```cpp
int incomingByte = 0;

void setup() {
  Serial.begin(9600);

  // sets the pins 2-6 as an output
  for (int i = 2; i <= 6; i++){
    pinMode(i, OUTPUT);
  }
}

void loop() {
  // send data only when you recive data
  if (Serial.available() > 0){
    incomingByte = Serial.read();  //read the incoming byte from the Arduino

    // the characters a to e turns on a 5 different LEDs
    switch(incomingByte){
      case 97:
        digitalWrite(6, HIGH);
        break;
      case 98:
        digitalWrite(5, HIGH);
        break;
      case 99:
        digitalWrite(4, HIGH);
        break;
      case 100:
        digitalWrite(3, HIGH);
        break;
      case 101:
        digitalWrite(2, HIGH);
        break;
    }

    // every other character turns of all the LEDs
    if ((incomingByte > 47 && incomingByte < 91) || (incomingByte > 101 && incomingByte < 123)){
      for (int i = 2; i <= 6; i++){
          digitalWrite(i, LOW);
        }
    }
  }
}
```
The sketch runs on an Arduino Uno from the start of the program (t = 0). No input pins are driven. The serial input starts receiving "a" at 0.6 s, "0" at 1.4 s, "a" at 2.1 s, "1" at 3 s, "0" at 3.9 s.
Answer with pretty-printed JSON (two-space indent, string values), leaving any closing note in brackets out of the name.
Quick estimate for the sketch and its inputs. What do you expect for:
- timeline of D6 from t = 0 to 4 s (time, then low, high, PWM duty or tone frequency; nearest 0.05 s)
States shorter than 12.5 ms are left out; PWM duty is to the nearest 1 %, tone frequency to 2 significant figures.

{
  "timeline of D6 from t = 0 to 4 s": "0 s low; 0.6 s high; 1.4 s low; 2.1 s high; 3 s low"
}
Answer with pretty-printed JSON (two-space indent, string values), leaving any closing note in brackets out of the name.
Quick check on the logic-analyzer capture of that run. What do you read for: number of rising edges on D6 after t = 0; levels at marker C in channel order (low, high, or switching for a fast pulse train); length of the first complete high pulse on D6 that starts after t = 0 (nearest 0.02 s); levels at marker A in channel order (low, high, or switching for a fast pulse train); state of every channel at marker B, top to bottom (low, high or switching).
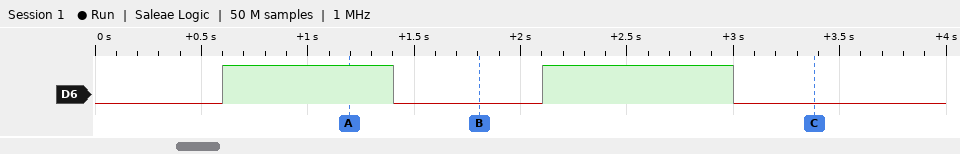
{
  "number of rising edges on D6 after t = 0": "2",
  "levels at marker C in channel order": "D6 low",
  "length of the first complete high pulse on D6 that starts after t = 0": "0.80 s",
  "levels at marker A in channel order": "D6 high",
  "state of every channel at marker B, top to bottom": "D6 low"
}
